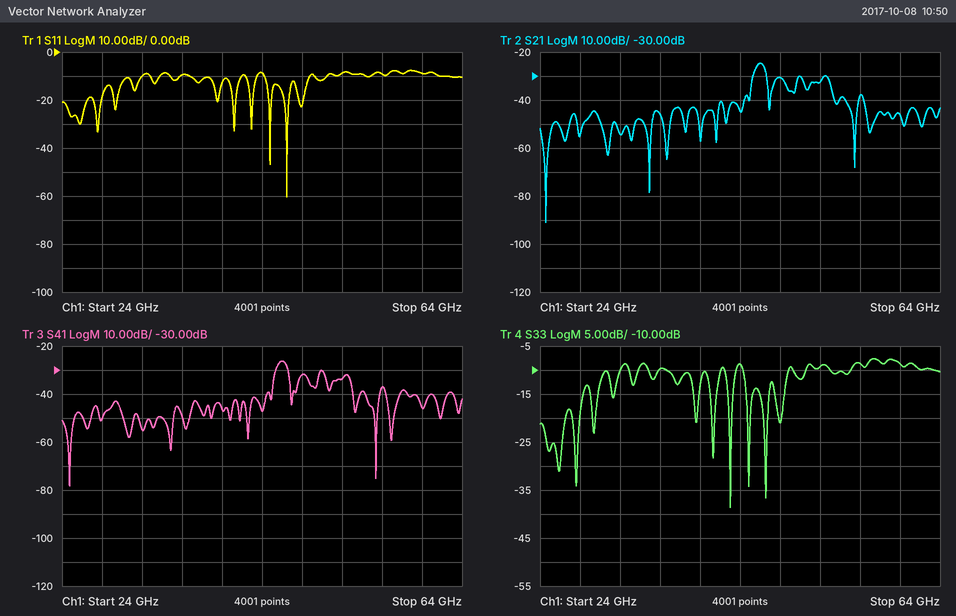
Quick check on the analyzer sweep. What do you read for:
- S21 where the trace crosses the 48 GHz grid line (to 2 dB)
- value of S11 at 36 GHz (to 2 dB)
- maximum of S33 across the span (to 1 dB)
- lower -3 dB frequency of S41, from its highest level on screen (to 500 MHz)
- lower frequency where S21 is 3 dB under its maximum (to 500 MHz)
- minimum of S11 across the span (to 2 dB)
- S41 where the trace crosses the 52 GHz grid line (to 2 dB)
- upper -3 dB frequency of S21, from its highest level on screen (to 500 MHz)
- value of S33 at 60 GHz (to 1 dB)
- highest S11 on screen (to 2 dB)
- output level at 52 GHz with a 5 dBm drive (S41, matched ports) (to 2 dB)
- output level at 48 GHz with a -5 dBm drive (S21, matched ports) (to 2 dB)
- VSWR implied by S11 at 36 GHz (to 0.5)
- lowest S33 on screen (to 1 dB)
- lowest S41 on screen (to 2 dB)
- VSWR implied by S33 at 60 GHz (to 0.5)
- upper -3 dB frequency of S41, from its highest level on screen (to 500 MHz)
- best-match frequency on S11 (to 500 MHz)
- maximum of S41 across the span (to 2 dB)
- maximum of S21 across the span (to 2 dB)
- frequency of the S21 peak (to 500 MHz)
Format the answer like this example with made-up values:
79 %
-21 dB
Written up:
-30 dB
-10 dB
-8 dB
45.5 GHz
45.5 GHz
-60 dB
-34 dB
46.5 GHz
-9 dB
-8 dB
-28 dBm
-36 dBm
2.0
-39 dB
-78 dB
2.0
46.5 GHz
46.5 GHz
-26 dB
-24 dB
46.0 GHz
